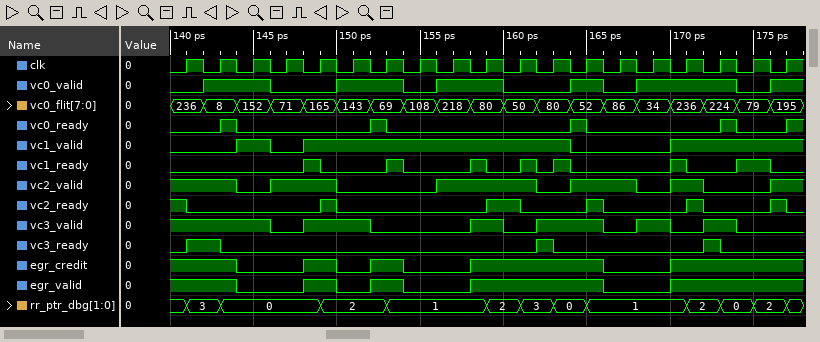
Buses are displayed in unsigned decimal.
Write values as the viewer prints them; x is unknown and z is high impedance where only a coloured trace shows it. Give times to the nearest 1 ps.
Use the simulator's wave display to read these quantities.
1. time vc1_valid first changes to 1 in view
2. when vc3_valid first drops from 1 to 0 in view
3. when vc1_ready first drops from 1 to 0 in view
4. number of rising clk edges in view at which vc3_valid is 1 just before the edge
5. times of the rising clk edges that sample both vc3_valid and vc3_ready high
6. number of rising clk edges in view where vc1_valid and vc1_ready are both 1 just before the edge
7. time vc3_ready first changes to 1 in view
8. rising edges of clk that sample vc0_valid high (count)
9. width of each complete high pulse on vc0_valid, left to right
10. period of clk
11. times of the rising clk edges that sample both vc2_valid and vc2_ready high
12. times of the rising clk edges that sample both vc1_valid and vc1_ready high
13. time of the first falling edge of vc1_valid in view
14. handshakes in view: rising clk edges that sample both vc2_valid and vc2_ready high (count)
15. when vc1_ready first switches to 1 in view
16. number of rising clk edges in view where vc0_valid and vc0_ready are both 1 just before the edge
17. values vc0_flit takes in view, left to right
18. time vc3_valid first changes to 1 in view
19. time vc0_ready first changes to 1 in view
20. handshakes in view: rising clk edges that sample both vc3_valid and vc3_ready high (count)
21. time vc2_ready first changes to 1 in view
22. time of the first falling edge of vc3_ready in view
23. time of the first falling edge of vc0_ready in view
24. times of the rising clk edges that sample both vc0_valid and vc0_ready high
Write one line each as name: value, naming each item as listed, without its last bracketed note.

time vc1_valid first changes to 1 in view: 144 ps
when vc3_valid first drops from 1 to 0 in view: 146 ps
when vc1_ready first drops from 1 to 0 in view: 149 ps
number of rising clk edges in view at which vc3_valid is 1 just before the edge: 10
times of the rising clk edges that sample both vc3_valid and vc3_ready high: 143 ps, 163 ps, 173 ps
number of rising clk edges in view where vc1_valid and vc1_ready are both 1 just before the edge: 4
time vc3_ready first changes to 1 in view: 141 ps
rising edges of clk that sample vc0_valid high: 11
width of each complete high pulse on vc0_valid, left to right: 4 ps, 4 ps, 4 ps, 2 ps, 6 ps
period of clk: 2 ps
times of the rising clk edges that sample both vc2_valid and vc2_ready high: 141 ps, 161 ps, 177 ps
times of the rising clk edges that sample both vc1_valid and vc1_ready high: 149 ps, 159 ps, 171 ps, 175 ps
time of the first falling edge of vc1_valid in view: 146 ps
handshakes in view: rising clk edges that sample both vc2_valid and vc2_ready high: 3
when vc1_ready first switches to 1 in view: 148 ps
number of rising clk edges in view where vc0_valid and vc0_ready are both 1 just before the edge: 2
values vc0_flit takes in view, left to right: 236, 8, 152, 71, 165, 143, 69, 108, 218, 80, 50, 80, 52, 86, 34, 236, 224, 79, 195
time vc3_valid first changes to 1 in view: 148 ps
time vc0_ready first changes to 1 in view: 143 ps
handshakes in view: rising clk edges that sample both vc3_valid and vc3_ready high: 3
time vc2_ready first changes to 1 in view: 149 ps
time of the first falling edge of vc3_ready in view: 143 ps
time of the first falling edge of vc0_ready in view: 144 ps
times of the rising clk edges that sample both vc0_valid and vc0_ready high: 153 ps, 165 ps
